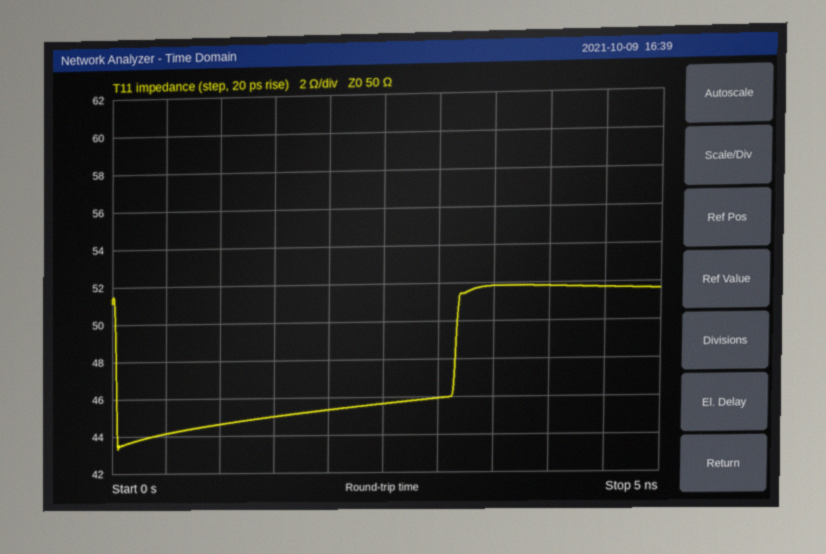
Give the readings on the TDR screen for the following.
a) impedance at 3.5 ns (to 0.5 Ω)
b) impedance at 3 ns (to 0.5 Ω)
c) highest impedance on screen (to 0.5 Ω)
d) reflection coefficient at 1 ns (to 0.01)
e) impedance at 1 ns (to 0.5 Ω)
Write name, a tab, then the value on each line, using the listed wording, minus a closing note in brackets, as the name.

impedance at 3.5 ns	52.0 Ω
impedance at 3 ns	46.0 Ω
highest impedance on screen	52.0 Ω
reflection coefficient at 1 ns	-0.06
impedance at 1 ns	44.5 Ω
